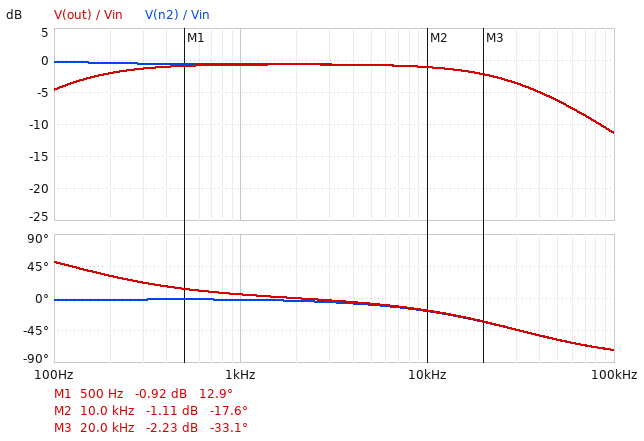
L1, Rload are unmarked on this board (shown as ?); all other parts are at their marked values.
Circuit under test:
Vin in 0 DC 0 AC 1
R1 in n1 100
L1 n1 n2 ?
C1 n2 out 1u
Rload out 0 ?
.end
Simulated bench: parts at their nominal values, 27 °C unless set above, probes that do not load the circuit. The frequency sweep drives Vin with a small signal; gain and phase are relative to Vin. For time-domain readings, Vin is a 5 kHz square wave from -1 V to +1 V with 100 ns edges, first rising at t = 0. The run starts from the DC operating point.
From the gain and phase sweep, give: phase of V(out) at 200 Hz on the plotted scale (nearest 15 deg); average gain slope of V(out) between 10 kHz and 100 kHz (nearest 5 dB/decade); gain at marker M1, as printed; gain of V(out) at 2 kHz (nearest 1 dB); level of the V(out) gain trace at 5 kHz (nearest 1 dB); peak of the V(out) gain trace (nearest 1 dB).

30 deg
-10 dB/decade
-0.92 dB
-1 dB
-1 dB
-1 dB
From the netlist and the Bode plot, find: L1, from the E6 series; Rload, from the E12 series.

6.8 mH
1.2 kΩ
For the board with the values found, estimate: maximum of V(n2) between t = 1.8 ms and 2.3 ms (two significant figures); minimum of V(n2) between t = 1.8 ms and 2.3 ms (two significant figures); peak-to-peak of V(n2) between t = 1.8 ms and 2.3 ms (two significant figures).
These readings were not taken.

920 mV
-950 mV
1.9 V
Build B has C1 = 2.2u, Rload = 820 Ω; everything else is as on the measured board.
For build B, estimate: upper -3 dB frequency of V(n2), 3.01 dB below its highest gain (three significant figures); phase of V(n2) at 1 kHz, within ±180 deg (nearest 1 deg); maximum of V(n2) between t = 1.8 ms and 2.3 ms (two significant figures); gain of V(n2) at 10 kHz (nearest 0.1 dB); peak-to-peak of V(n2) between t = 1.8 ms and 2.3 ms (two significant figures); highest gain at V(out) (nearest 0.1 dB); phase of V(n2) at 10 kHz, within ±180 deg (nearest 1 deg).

16.6 kHz
-3 deg
860 mV
-1.8 dB
1.8 V
-1.0 dB
-25 deg
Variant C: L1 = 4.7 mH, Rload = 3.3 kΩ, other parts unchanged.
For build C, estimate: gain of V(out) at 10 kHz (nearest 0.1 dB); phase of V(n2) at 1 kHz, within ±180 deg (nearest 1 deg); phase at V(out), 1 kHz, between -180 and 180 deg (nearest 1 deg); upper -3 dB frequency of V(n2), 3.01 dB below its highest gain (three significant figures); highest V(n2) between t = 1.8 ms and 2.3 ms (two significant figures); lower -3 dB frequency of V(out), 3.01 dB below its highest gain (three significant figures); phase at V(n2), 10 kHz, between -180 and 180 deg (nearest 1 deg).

-0.3 dB
-1 deg
2 deg
108 kHz
960 mV
46.8 Hz
-5 deg
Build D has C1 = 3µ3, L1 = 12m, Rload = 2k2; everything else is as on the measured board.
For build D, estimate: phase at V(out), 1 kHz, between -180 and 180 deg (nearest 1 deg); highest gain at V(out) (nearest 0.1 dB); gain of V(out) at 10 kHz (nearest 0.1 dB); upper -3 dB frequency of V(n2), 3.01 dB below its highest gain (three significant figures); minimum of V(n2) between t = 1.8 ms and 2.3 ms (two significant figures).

-1 deg
-0.4 dB
-0.8 dB
27.8 kHz
-990 mV
